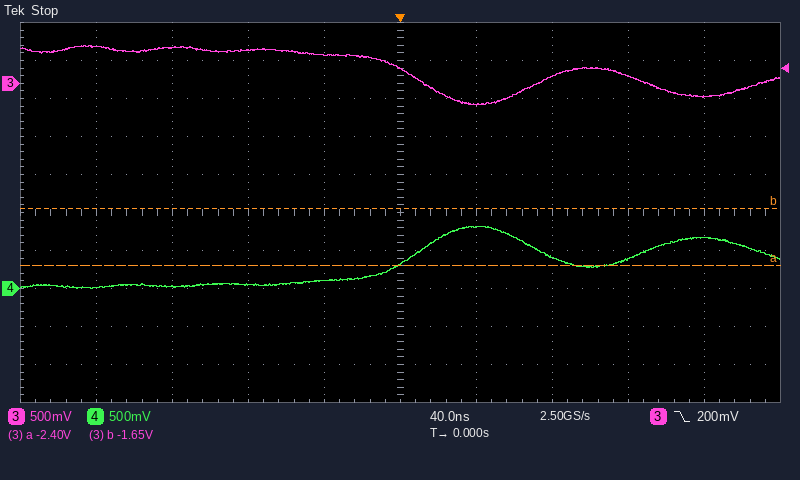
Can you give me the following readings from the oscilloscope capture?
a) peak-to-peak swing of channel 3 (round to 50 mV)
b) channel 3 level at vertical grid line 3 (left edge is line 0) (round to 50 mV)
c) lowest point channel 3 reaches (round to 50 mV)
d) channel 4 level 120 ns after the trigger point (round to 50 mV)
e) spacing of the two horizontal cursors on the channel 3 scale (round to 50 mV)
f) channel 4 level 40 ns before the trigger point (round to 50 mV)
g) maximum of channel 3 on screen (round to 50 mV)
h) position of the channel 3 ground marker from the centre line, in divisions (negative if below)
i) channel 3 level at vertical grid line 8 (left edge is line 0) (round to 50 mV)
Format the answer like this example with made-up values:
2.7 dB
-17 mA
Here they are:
800 mV
450 mV
-300 mV
400 mV
750 mV
100 mV
500 mV
+3.4 div
100 mV
